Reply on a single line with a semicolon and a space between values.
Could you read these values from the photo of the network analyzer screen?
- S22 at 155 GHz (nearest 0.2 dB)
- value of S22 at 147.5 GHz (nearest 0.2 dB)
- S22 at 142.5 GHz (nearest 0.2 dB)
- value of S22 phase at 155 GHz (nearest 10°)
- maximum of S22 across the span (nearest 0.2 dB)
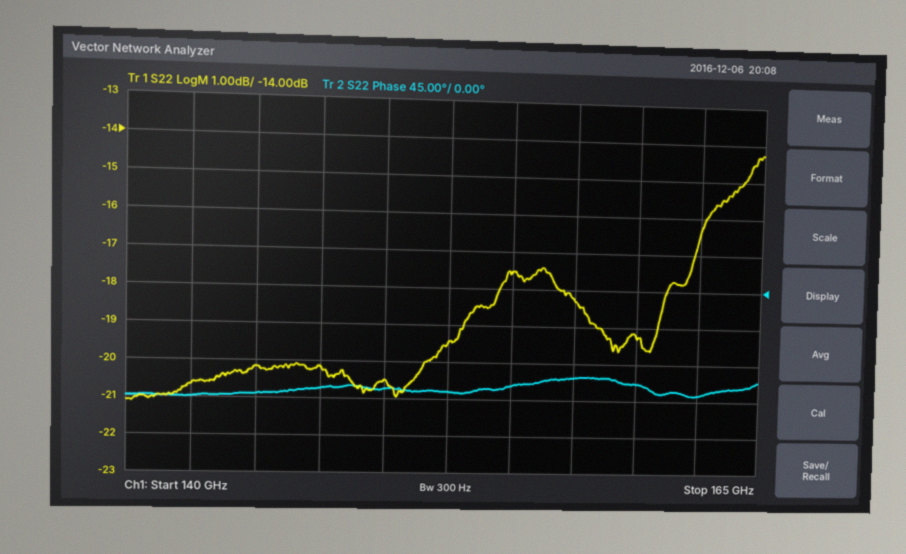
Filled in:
-17.6 dB; -20.2 dB; -20.6 dB; -120°; -14.2 dB
